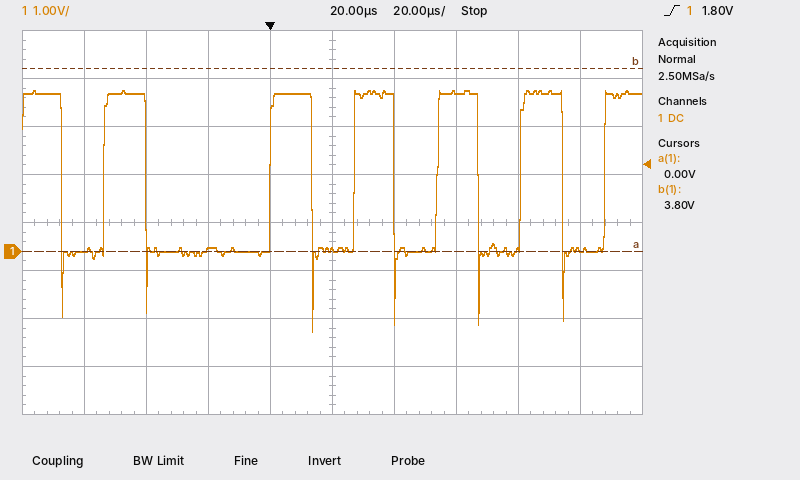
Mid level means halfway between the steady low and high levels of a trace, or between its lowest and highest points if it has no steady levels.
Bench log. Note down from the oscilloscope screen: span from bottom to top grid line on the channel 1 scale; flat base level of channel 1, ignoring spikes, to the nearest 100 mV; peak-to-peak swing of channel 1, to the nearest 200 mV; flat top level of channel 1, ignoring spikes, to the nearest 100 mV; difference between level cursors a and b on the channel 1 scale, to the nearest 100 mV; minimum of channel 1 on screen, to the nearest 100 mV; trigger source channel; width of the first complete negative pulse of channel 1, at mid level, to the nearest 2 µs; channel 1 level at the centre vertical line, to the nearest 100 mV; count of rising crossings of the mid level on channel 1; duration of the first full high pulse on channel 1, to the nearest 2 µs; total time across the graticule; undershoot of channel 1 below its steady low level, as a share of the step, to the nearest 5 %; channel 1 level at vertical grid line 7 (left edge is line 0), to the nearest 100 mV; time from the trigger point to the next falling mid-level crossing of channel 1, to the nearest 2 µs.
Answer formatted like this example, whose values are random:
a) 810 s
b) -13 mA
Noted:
a) 8 V
b) 0.0 V
c) 5.0 V
d) 3.3 V
e) 3.8 V
f) -1.7 V
g) channel 1
h) 14 µs
i) 0.0 V
j) 6
k) 14 µs
l) 200 µs
m) 50 %
n) 3.3 V
o) 14 µs
